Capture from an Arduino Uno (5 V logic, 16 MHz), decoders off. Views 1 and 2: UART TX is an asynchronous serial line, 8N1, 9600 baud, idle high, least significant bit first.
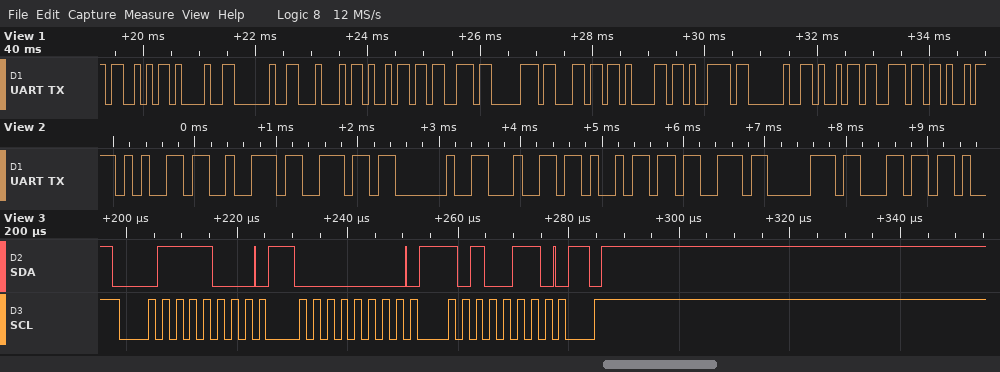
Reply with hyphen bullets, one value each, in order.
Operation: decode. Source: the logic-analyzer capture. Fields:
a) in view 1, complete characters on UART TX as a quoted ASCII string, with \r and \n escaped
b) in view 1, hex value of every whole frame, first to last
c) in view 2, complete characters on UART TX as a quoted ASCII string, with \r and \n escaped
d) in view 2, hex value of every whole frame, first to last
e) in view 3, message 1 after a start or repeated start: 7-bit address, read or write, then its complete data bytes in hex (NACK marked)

- "S! Display in"
- 0x53 0x21 0x20 0x44 0x69 0x73 0x70 0x6C 0x61 0x79 0x20 0x69 0x6E
- "ern displ"
- 65 72 6E 20 64 69 73 70 6C
- 0x3C write: 00 A6
